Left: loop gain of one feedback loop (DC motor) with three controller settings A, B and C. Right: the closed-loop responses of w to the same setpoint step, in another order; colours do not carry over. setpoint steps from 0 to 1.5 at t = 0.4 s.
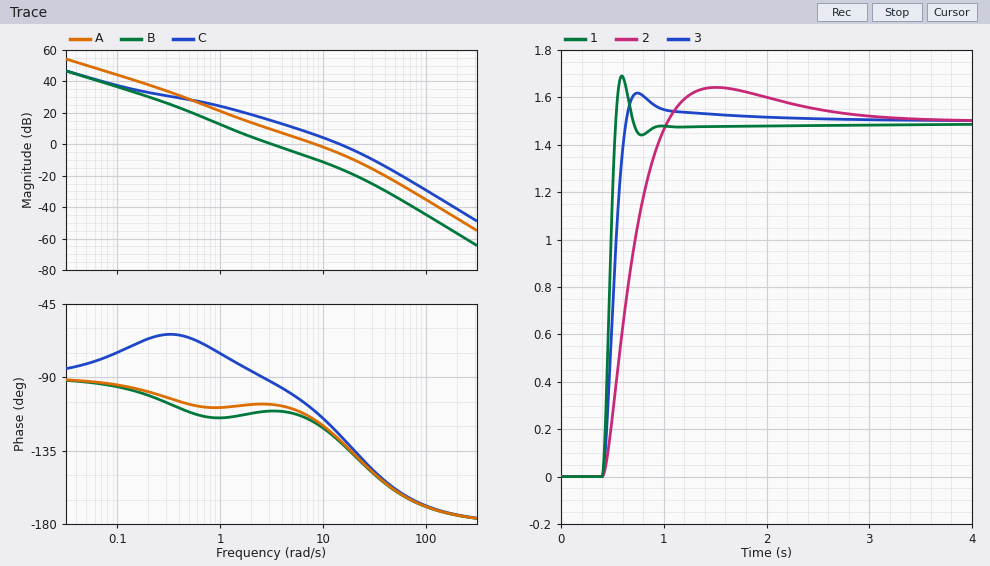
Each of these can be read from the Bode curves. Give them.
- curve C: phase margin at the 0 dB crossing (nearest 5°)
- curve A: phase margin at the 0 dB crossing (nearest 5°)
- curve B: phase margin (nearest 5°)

55°
65°
70°
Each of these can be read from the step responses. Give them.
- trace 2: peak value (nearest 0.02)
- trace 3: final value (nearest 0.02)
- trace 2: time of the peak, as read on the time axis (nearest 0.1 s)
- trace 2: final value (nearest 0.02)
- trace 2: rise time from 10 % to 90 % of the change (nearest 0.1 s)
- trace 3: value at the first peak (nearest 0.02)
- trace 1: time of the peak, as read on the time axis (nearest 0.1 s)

1.64
1.50
1.5 s
1.50
0.4 s
1.62
0.6 s
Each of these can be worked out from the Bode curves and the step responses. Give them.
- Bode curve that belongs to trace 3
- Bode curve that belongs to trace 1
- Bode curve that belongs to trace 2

A
C
B
